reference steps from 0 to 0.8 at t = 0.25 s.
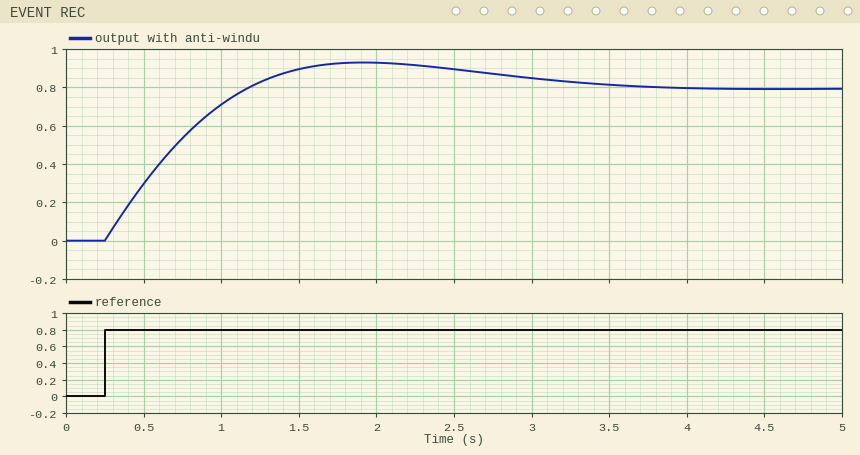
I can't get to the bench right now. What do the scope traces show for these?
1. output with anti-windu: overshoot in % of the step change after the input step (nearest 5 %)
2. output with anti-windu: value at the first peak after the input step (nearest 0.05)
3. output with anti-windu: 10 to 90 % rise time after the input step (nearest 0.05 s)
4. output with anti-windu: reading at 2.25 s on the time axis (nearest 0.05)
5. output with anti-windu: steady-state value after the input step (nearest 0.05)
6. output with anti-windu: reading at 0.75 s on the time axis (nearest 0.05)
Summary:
15 %
0.95
0.70 s
0.90
0.80
0.55
